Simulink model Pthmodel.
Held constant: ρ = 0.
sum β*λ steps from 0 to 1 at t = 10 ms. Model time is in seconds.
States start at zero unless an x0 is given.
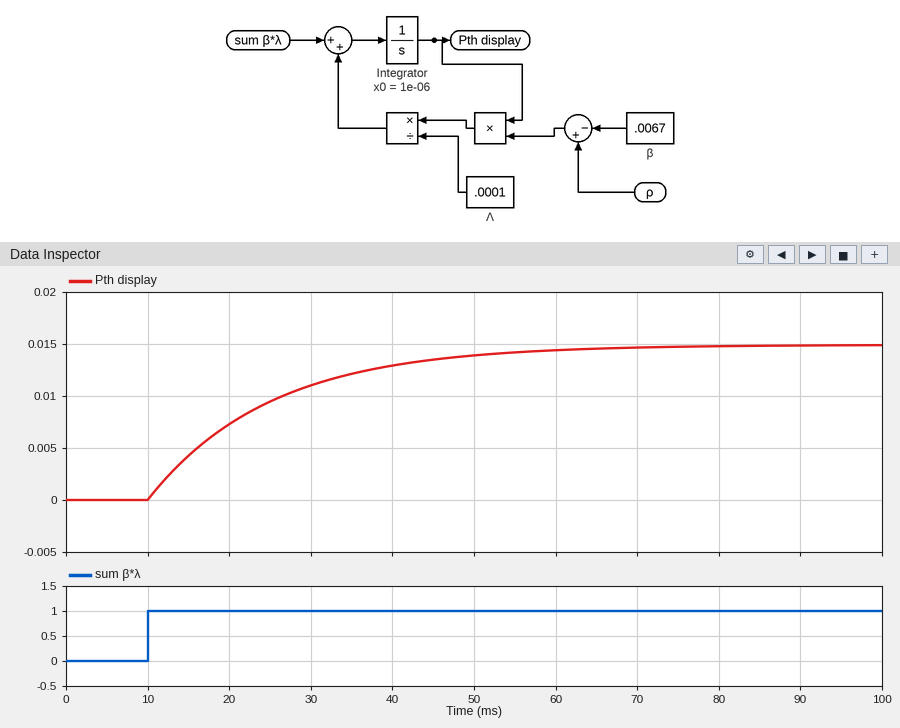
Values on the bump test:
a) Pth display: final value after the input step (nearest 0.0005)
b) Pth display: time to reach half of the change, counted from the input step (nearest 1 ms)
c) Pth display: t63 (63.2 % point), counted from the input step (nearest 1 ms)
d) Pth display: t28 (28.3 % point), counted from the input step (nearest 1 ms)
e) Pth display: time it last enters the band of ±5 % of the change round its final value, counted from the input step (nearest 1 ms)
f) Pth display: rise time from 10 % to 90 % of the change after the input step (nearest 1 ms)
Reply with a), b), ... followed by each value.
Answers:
a) 0.0150
b) 10 ms
c) 15 ms
d) 5 ms
e) 45 ms
f) 33 ms
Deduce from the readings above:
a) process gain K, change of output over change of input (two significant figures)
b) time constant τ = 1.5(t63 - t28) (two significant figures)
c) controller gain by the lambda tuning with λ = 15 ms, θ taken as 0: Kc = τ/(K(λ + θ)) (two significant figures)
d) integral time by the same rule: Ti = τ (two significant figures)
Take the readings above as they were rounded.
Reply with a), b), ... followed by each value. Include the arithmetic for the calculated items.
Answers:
a) (0.015 - 0) / 1 = 0.015
b) 1.5 × (15 - 5) = 15 ms
c) 15 / (0.015 × (15 + 0)) = 67
d) 15 ms
